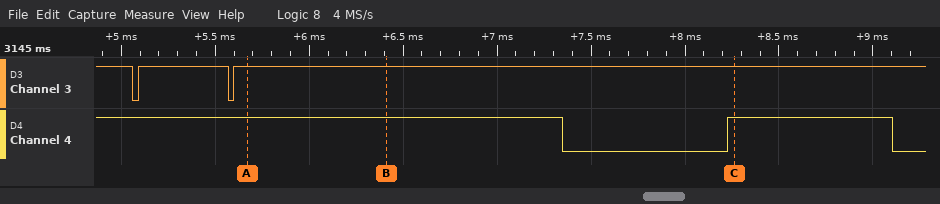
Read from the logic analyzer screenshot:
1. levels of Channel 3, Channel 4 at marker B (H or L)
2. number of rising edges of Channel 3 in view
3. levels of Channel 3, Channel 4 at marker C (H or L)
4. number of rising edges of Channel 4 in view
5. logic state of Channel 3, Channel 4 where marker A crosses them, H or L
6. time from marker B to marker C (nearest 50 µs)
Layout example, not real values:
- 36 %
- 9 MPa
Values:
- Channel 3=H, Channel 4=H
- 2
- Channel 3=H, Channel 4=H
- 1
- Channel 3=H, Channel 4=H
- 1850 µs
